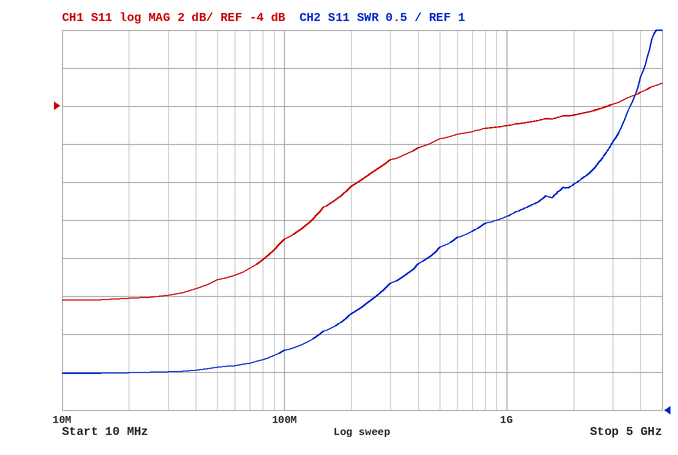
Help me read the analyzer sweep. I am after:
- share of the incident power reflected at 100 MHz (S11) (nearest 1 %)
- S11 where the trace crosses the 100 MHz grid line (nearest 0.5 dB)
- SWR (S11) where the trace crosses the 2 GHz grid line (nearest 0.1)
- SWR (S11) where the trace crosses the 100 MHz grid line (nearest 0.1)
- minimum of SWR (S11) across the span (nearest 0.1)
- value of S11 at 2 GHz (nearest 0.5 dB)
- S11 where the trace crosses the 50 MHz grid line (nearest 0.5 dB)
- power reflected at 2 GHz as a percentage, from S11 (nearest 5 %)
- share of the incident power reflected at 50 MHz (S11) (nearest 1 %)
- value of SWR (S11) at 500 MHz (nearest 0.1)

8 %
-11.0 dB
4.0
1.8
1.5
-4.5 dB
-13.0 dB
35 %
5 %
3.1
